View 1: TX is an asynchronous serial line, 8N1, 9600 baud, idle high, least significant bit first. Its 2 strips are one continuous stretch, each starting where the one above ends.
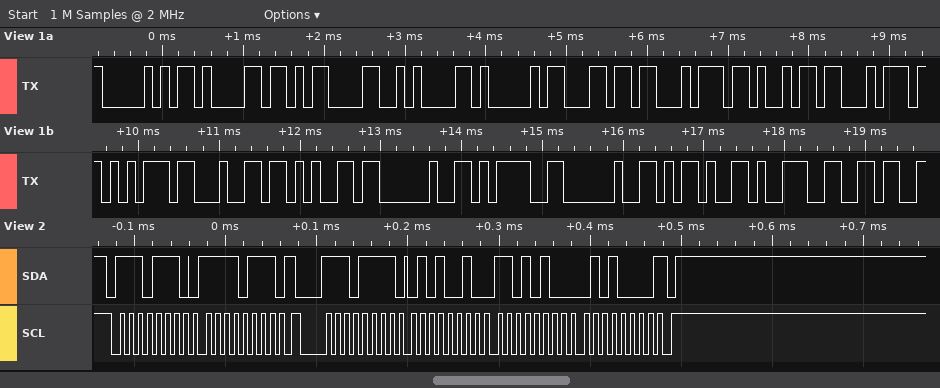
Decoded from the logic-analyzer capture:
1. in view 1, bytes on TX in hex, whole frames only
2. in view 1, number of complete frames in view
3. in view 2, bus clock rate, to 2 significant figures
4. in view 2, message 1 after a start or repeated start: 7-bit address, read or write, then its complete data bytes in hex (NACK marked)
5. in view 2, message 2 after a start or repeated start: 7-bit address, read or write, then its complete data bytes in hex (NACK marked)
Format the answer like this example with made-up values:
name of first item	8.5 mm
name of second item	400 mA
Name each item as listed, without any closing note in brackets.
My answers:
in view 1, bytes on TX in hex, whole frames only	50 61 0D 0A 41 6C 74 69 74 75 64 65 20 3D 20 2D 39 36
in view 1, number of complete frames in view	18
in view 2, bus clock rate, to 2 significant figures	100 kHz
in view 2, message 1 after a start or repeated start: 7-bit address, read or write, then its complete data bytes in hex	0x77 write: F7
in view 2, message 2 after a start or repeated start: 7-bit address, read or write, then its complete data bytes in hex	0x77 read: 52 D4 50 NACK
